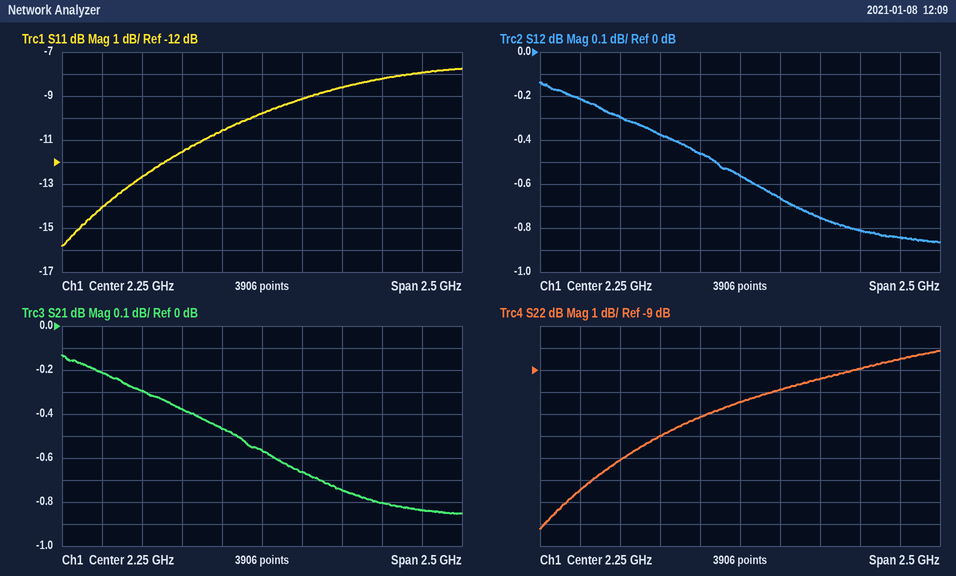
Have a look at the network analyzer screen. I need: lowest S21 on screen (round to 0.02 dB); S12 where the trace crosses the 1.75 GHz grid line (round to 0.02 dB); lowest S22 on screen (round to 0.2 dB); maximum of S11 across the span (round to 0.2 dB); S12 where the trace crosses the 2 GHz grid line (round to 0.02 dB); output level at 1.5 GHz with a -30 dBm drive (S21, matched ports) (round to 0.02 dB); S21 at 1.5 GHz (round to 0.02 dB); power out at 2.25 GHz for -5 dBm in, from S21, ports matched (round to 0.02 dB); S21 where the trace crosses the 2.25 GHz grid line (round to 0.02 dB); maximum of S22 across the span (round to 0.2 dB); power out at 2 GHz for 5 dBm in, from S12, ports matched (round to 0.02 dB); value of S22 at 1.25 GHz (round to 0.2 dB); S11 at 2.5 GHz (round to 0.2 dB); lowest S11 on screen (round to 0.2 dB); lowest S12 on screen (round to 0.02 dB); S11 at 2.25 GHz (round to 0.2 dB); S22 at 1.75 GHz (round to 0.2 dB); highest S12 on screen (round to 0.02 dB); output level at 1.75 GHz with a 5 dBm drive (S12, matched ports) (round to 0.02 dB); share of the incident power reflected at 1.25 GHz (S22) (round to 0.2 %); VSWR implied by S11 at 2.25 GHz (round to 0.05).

-0.86 dB
-0.38 dB
-16.2 dB
-7.8 dB
-0.46 dB
-30.30 dBm
-0.30 dB
-5.56 dBm
-0.56 dB
-8.2 dB
4.54 dBm
-14.4 dB
-9.2 dB
-15.8 dB
-0.86 dB
-9.8 dB
-12.0 dB
-0.14 dB
4.62 dBm
3.6 %
1.95
